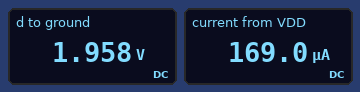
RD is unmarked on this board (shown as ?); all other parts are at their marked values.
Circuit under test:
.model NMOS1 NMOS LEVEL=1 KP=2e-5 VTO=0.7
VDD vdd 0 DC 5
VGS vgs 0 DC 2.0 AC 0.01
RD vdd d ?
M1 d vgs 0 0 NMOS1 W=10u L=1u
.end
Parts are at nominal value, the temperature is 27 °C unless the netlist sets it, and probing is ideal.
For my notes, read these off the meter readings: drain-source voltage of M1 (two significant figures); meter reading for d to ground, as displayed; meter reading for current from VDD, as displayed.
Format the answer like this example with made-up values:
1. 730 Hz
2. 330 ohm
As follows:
1. 2.0 V
2. 1.958 V
3. 169.0 µA
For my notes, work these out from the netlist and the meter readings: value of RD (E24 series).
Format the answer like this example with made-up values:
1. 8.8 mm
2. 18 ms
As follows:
1. 18 kΩ
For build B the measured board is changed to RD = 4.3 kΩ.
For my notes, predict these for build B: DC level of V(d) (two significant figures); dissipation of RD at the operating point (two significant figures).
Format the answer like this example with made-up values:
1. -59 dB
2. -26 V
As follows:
1. 4.3 V
2. 120 µW
